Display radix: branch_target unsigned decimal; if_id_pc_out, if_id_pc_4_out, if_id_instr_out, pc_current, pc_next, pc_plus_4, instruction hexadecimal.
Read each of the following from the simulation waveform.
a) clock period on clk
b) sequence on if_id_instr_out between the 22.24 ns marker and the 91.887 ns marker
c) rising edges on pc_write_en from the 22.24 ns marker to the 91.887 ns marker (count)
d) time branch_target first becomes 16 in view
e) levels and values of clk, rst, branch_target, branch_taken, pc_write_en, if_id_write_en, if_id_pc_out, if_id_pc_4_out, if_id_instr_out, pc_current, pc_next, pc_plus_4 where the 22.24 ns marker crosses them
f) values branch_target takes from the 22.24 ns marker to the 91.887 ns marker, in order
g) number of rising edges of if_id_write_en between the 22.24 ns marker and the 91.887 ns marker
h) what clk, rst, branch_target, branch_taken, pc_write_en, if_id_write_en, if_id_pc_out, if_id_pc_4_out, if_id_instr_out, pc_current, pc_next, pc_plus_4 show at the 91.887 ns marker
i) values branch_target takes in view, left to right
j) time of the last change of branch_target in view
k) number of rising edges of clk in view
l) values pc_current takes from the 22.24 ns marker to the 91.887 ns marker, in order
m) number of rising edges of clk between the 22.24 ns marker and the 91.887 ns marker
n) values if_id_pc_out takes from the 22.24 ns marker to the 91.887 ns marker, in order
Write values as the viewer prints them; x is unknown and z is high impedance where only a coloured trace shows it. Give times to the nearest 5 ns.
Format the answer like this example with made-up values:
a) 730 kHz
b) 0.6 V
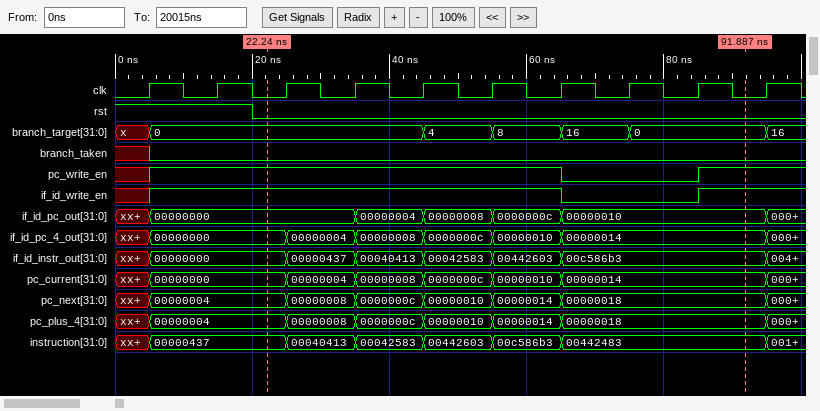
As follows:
a) 10 ns
b) 00000000, 00000437, 00040413, 00042583, 00442603, 00c586b3
c) 1
d) 65 ns
e) clk=0, rst=0, branch_target=0, branch_taken=0, pc_write_en=1, if_id_write_en=1, if_id_pc_out=00000000, if_id_pc_4_out=00000000, if_id_instr_out=00000000, pc_current=00000000, pc_next=00000004, pc_plus_4=00000004
f) 0, 4, 8, 16, 0
g) 1
h) clk=0, rst=0, branch_target=0, branch_taken=0, pc_write_en=1, if_id_write_en=1, if_id_pc_out=00000010, if_id_pc_4_out=00000014, if_id_instr_out=00c586b3, pc_current=00000014, pc_next=00000018, pc_plus_4=00000018
i) x, 0, 4, 8, 16, 0, 16
j) 95 ns
k) 10
l) 00000000, 00000004, 00000008, 0000000c, 00000010, 00000014
m) 7
n) 00000000, 00000004, 00000008, 0000000c, 00000010
